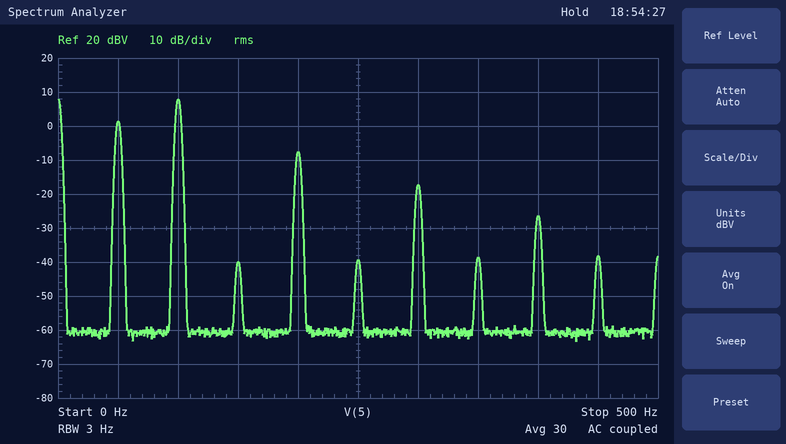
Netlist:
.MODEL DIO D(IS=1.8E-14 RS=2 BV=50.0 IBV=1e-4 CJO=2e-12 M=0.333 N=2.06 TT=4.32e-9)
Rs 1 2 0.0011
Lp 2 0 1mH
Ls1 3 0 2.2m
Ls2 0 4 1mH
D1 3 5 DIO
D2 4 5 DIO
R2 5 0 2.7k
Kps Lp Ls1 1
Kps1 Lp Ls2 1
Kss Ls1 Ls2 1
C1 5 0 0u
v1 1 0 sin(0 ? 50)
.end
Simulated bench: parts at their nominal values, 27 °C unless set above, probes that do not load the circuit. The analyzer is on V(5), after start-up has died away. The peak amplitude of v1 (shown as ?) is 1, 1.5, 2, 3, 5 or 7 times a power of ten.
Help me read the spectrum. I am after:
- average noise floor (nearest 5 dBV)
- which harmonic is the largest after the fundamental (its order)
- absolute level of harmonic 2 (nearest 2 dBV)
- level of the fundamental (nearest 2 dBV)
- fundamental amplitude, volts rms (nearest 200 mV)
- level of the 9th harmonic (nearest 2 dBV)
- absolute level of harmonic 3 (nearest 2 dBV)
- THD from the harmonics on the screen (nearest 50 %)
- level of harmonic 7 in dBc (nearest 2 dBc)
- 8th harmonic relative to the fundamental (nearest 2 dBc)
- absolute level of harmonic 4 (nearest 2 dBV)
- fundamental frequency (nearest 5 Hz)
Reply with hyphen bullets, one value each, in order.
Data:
- -60 dBV
- 2
- 8 dBV
- 2 dBV
- 1.2 V
- -38 dBV
- -40 dBV
- 200 %
- -40 dBc
- -28 dBc
- -8 dBV
- 50 Hz
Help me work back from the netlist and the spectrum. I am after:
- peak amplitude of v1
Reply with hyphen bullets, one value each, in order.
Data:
- 7 V
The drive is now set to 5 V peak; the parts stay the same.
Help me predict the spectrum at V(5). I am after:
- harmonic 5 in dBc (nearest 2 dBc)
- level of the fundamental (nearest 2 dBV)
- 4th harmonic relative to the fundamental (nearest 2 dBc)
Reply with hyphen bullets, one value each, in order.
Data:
- -34 dBc
- -2 dBV
- -10 dBc
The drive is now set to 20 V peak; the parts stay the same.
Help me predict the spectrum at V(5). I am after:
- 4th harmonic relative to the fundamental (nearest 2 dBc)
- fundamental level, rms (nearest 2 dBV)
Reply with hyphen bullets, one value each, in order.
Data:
- -8 dBc
- 10 dBV
